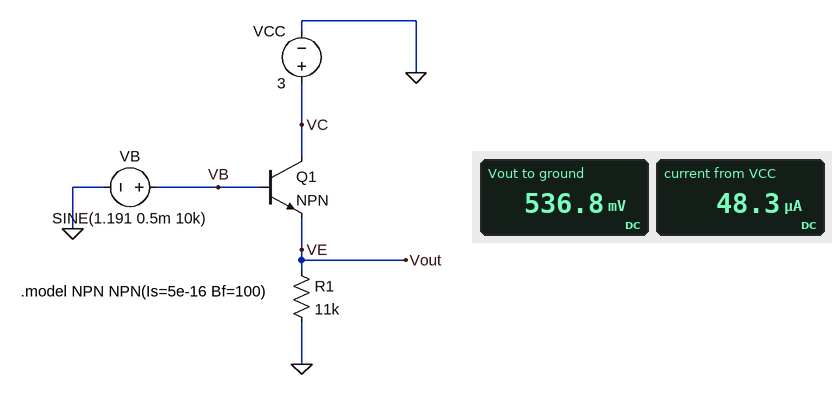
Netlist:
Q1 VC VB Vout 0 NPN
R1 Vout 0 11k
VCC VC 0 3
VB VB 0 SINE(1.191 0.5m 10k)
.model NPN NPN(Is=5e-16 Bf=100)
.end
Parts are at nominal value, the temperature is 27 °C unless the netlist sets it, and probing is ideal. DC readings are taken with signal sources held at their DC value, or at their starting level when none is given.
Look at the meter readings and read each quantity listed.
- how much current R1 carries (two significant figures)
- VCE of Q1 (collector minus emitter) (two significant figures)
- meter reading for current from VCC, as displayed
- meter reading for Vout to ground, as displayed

49 µA
2.5 V
48.3 µA
536.8 mV
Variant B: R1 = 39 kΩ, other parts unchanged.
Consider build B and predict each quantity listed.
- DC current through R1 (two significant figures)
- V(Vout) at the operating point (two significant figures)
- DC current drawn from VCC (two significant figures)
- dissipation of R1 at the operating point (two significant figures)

15 µA
570 mV
14 µA
8.3 µW
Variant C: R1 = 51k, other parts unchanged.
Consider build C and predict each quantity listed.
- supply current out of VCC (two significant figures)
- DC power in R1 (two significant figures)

11 µA
6.5 µW
